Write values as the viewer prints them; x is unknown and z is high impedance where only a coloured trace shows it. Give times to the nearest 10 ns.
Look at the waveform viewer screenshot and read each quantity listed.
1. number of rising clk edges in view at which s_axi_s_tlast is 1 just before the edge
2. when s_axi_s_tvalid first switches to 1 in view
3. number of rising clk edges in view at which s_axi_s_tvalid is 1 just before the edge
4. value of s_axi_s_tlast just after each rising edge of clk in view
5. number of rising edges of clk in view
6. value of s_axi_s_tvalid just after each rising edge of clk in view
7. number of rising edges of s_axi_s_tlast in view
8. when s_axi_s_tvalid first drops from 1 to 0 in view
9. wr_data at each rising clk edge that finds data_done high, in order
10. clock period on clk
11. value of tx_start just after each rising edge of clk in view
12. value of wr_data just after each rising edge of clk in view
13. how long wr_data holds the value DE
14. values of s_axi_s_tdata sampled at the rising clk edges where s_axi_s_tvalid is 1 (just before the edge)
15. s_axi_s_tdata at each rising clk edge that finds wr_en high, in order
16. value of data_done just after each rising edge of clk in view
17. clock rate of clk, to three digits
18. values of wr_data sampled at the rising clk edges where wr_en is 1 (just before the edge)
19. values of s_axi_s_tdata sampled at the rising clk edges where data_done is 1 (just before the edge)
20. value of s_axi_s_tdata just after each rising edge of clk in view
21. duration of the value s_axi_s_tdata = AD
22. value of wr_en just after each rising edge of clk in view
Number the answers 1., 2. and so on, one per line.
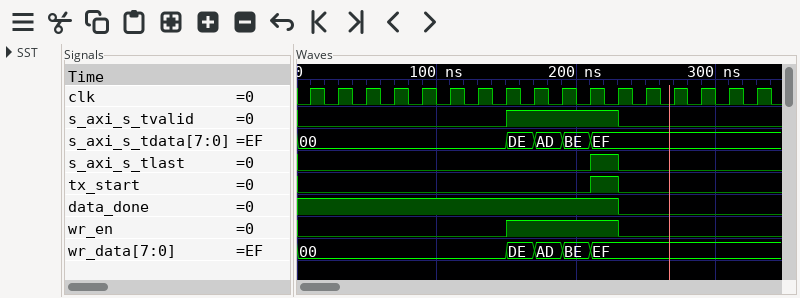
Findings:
1. 1
2. 150 ns
3. 4
4. 0 0 0 0 0 0 0 0 0 0 1 0 0 0 0 0 0
5. 17
6. 0 0 0 0 0 0 0 1 1 1 1 0 0 0 0 0 0
7. 1
8. 230 ns
9. 00, 00, 00, 00, 00, 00, 00, 00, DE, AD, BE, EF
10. 20 ns
11. 0 0 0 0 0 0 0 0 0 0 1 0 0 0 0 0 0
12. 00, 00, 00, 00, 00, 00, 00, DE, AD, BE, EF, EF, EF, EF, EF, EF, EF
13. 20 ns
14. DE, AD, BE, EF
15. DE, AD, BE, EF
16. 1 1 1 1 1 1 1 1 1 1 1 0 0 0 0 0 0
17. 50.0 MHz
18. DE, AD, BE, EF
19. 00, 00, 00, 00, 00, 00, 00, 00, DE, AD, BE, EF
20. 00, 00, 00, 00, 00, 00, 00, DE, AD, BE, EF, EF, EF, EF, EF, EF, EF
21. 20 ns
22. 0 0 0 0 0 0 0 1 1 1 1 0 0 0 0 0 0
